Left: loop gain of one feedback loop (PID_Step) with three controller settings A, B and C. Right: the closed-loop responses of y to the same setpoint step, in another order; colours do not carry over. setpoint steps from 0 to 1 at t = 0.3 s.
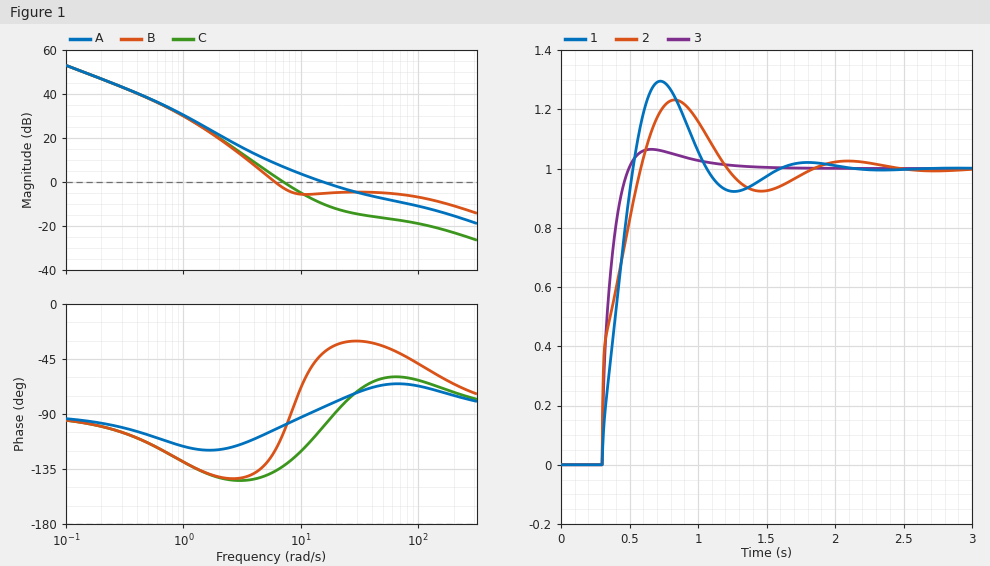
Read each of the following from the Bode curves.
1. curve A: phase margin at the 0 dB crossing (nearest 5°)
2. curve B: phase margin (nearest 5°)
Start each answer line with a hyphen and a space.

- 95°
- 60°
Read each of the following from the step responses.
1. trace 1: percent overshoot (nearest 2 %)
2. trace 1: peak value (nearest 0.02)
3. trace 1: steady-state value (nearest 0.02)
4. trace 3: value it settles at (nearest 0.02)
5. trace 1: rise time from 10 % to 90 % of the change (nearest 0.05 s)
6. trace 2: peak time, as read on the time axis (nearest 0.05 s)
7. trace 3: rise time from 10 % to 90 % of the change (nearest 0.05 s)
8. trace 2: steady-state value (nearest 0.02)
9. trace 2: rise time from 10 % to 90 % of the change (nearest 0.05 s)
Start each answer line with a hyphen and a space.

- 30 %
- 1.30
- 1.00
- 1.00
- 0.20 s
- 0.85 s
- 0.15 s
- 1.00
- 0.25 s
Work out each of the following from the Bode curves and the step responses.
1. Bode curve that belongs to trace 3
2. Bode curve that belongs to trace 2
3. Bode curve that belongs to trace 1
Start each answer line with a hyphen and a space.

- A
- B
- C
